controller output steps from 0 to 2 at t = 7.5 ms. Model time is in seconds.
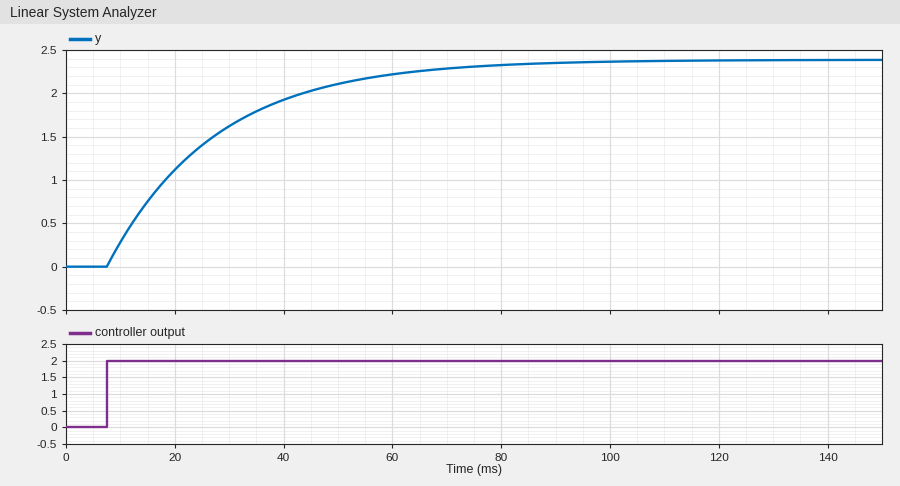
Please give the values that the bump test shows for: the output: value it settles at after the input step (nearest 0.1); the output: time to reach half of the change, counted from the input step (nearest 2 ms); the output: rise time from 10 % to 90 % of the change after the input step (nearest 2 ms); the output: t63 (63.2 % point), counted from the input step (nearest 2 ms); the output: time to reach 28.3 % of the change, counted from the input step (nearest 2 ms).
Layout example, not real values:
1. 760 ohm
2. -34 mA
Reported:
1. 2.4
2. 14 ms
3. 44 ms
4. 20 ms
5. 6 ms
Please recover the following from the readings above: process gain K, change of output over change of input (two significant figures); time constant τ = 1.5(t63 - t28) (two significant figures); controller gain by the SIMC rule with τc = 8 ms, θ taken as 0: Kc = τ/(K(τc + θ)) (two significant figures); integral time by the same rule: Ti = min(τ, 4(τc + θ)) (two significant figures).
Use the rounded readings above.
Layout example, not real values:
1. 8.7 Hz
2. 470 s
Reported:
1. 1.2
2. 21 ms
3. 2.2
4. 21 ms
